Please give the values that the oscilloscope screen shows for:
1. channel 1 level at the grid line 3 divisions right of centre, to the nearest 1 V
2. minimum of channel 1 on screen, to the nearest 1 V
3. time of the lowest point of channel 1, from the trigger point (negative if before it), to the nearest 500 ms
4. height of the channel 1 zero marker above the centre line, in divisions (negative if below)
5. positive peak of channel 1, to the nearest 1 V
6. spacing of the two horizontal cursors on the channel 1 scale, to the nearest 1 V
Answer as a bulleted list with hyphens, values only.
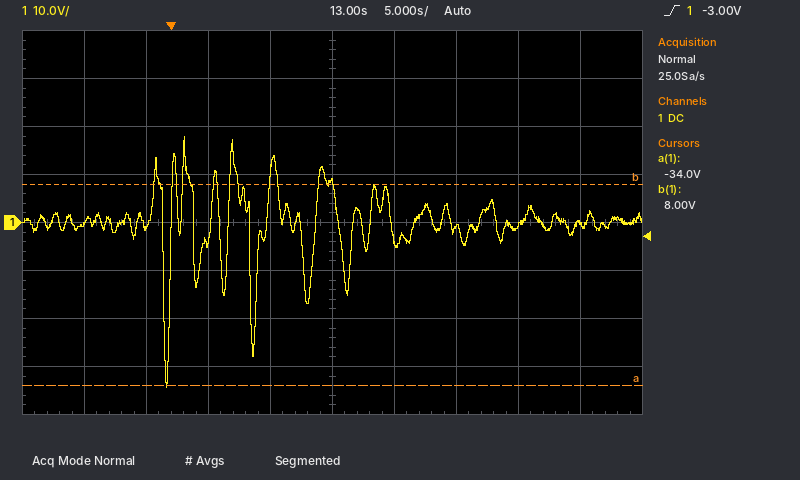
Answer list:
- -1 V
- -34 V
- -500 ms
- 0.0 div
- 18 V
- 42 V
